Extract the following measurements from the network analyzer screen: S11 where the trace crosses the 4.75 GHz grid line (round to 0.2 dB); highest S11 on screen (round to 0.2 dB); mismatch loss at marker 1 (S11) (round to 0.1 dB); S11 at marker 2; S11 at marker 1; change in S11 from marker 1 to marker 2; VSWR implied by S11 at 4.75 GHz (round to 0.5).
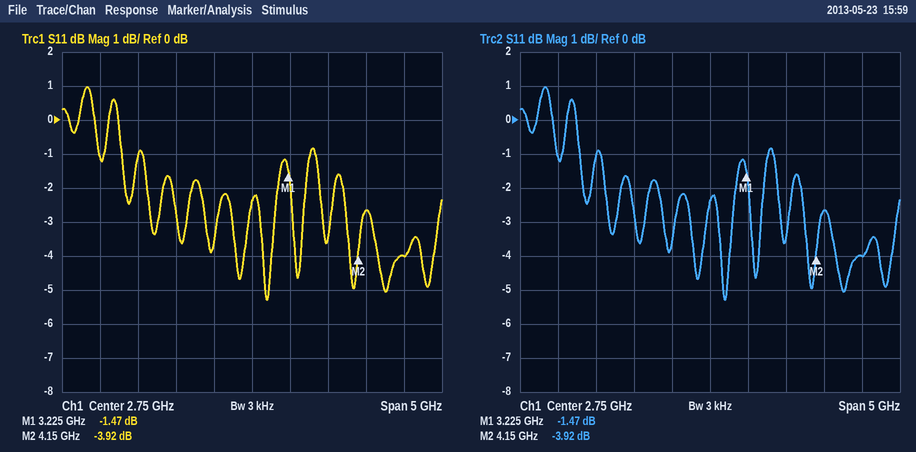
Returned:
-4.0 dB
1.0 dB
5.4 dB
-3.92 dB
-1.47 dB
-2.45 dB
4.5
